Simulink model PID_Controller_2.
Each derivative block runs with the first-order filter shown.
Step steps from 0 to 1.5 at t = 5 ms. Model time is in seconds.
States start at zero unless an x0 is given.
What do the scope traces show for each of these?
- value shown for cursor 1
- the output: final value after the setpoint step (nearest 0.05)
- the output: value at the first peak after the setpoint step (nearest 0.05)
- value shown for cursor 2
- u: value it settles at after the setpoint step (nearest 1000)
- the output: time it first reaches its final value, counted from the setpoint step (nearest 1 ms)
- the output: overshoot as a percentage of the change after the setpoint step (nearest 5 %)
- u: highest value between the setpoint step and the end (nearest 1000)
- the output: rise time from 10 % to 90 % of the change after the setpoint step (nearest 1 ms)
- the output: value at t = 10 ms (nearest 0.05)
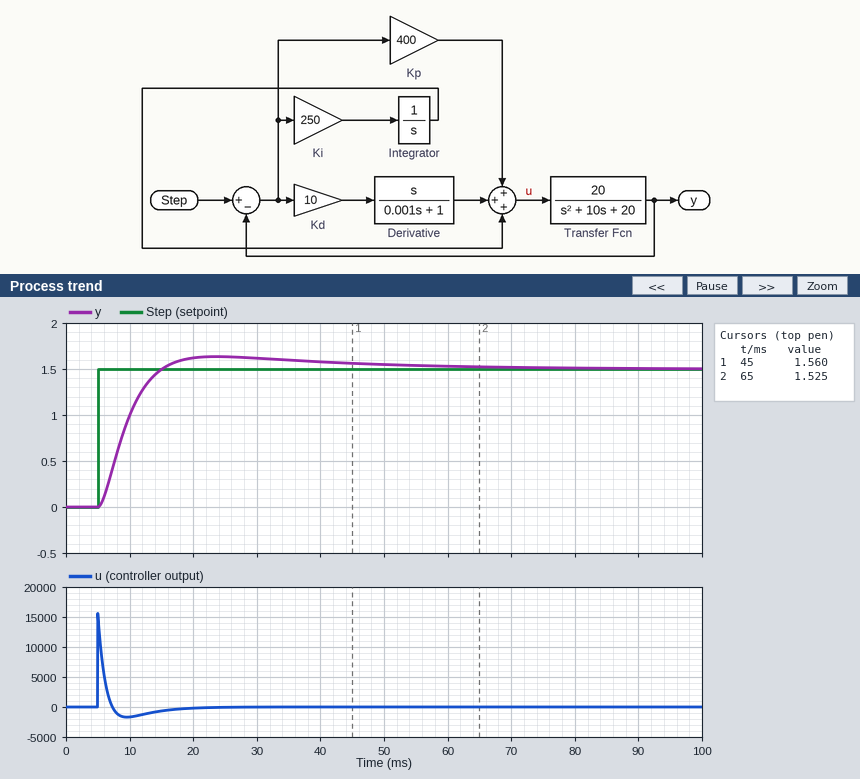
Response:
1.560
1.50
1.65
1.525
0
10 ms
10 %
16000
7 ms
1.00
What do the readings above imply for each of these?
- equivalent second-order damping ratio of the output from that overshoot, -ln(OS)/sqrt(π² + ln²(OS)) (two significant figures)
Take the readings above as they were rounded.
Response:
0.59
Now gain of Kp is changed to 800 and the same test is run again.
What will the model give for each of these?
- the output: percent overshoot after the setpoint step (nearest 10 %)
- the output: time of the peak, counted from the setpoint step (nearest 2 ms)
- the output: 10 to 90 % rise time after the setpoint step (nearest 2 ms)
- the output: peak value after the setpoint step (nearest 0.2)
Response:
20 %
14 ms
6 ms
1.8
